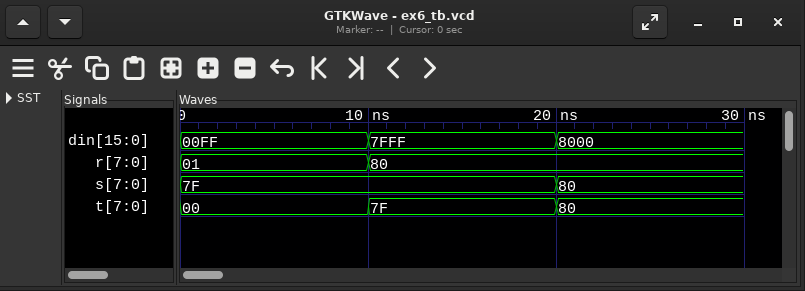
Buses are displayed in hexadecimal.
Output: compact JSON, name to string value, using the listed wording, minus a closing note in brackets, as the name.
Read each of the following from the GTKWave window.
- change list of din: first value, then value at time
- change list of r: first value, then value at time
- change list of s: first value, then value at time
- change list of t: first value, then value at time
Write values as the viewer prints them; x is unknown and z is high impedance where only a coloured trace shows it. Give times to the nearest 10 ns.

{"change list of din: first value, then value at time": "00FF, 7FFF at 10 ns, 8000 at 20 ns", "change list of r: first value, then value at time": "01, 80 at 10 ns", "change list of s: first value, then value at time": "7F, 80 at 20 ns", "change list of t: first value, then value at time": "00, 7F at 10 ns, 80 at 20 ns"}
